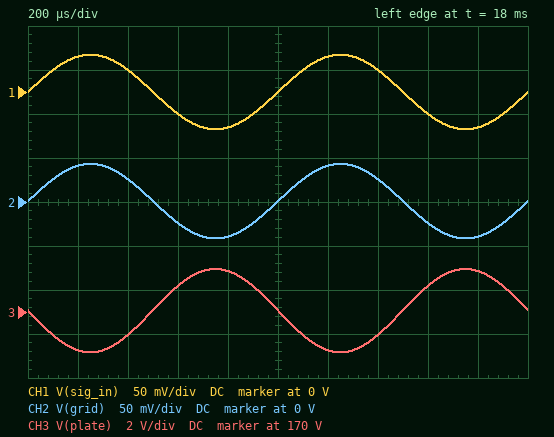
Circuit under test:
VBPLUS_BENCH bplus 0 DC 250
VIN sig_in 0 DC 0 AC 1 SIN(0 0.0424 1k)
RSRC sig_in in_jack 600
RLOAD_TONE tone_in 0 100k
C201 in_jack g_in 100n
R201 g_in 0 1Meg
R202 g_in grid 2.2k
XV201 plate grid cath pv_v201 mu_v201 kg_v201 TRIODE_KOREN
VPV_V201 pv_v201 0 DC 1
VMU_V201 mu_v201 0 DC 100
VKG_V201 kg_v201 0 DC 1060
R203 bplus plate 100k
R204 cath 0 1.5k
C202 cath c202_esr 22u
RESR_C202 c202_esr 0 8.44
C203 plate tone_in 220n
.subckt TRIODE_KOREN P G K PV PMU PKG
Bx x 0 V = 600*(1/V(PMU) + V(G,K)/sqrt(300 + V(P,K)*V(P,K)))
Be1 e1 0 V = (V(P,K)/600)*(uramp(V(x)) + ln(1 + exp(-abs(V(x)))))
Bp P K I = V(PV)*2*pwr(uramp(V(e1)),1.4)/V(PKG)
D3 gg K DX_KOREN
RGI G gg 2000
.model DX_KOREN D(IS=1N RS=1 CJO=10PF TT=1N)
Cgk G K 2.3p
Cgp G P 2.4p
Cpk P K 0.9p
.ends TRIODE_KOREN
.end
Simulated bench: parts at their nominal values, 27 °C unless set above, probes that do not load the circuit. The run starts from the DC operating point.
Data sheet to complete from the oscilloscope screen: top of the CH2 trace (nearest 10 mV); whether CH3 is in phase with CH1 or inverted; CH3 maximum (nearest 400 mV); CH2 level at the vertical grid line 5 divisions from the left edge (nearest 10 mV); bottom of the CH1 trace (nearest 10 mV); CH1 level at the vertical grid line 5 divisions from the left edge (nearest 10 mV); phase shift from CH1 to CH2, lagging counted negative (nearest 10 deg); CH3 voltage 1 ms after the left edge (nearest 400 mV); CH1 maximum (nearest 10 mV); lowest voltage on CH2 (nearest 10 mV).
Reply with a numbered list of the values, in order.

1. 40 mV
2. inverted
3. 172.0 V
4. 0 V
5. -40 mV
6. 0 V
7. 0 deg
8. 170.0 V
9. 40 mV
10. -40 mV
